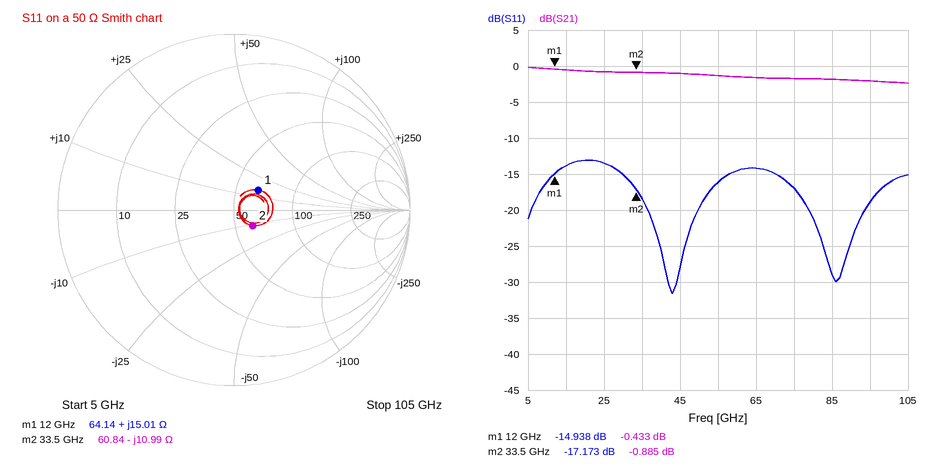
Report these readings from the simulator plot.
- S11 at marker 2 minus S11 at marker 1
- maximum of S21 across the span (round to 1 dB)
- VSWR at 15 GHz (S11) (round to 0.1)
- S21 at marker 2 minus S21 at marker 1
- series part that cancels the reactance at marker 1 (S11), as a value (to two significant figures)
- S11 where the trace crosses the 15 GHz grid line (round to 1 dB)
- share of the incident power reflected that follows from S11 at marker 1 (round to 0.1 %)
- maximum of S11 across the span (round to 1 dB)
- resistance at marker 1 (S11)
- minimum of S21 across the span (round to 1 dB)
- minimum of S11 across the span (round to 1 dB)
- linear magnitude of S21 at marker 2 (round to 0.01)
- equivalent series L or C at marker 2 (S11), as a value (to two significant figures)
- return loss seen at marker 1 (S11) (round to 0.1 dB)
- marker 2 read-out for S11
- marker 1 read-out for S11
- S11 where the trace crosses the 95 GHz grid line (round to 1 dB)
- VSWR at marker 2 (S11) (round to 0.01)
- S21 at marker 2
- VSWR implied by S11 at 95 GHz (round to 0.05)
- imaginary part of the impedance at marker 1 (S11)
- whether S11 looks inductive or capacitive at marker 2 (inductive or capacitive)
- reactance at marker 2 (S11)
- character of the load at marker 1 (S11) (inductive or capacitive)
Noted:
-2.235 dB
0 dB
1.5
-0.452 dB
880 fF
-14 dB
3.2 %
-13 dB
64.14 Ω
-2 dB
-32 dB
0.90
430 fF
14.9 dB
-17.173 dB
-14.938 dB
-19 dB
1.32
-0.885 dB
1.25
+15.01 Ω
capacitive
-10.99 Ω
inductive
